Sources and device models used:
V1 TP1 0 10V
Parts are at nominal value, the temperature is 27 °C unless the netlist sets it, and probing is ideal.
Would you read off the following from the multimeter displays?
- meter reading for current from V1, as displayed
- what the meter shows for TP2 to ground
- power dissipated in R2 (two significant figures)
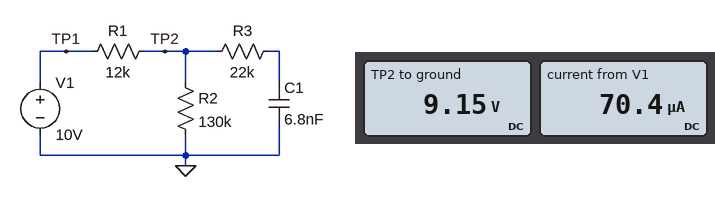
70.4 µA
9.15 V
640 µW
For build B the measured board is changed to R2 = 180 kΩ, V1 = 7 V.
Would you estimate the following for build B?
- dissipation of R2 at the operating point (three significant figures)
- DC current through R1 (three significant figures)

239 µW
36.5 µA
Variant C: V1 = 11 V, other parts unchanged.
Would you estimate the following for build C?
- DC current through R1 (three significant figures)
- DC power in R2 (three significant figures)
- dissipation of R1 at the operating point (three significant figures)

77.5 µA
780 µW
72.0 µW
